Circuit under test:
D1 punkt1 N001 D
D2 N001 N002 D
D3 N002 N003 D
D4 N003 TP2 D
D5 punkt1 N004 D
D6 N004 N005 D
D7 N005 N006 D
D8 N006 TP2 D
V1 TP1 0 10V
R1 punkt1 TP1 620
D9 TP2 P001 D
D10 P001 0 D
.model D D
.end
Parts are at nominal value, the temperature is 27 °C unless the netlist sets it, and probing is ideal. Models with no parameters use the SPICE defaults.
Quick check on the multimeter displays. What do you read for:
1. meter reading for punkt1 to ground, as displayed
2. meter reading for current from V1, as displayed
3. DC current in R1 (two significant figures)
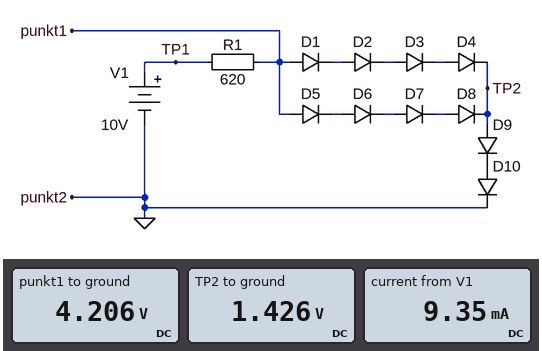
4.206 V
9.35 mA
9.3 mA
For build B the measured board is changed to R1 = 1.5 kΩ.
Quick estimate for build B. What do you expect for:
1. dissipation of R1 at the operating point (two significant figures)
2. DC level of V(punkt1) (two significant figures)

23 mW
4.1 V
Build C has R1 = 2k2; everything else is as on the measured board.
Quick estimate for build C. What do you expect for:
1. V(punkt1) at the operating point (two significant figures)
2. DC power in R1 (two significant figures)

4.0 V
16 mW
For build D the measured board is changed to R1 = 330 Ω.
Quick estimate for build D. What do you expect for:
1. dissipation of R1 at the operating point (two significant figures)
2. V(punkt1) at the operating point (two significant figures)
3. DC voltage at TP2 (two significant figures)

98 mW
4.3 V
1.5 V
